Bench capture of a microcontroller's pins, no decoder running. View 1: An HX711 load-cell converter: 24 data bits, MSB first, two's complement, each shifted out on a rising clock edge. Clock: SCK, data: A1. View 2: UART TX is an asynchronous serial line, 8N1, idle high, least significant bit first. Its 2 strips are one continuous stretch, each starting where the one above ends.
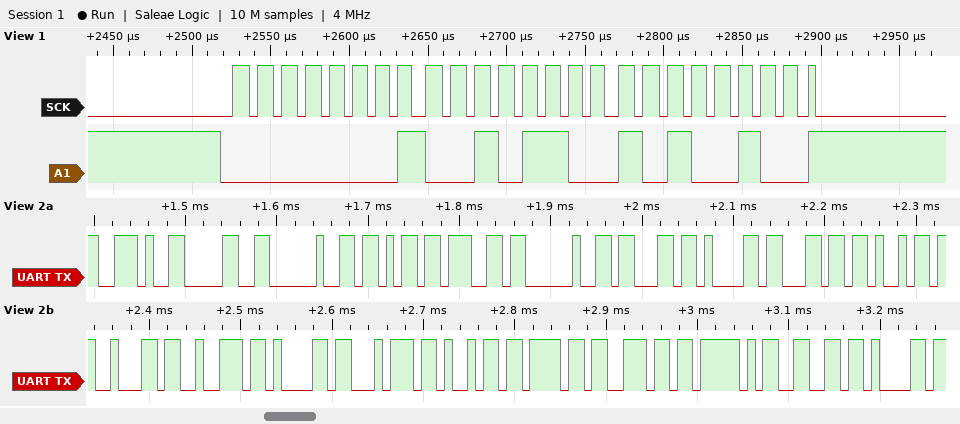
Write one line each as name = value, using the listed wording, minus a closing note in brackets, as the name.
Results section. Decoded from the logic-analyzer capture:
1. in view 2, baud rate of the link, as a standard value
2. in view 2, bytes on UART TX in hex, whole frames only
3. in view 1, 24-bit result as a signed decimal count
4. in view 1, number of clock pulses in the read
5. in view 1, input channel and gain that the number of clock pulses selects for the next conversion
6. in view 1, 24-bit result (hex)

in view 2, baud rate of the link, as a standard value = 115200 baud
in view 2, bytes on UART TX in hex, whole frames only = 0x2E 0x30 0x20 0x6B 0x67 0x20 0x63 0x61 0x6C 0x69 0x62 0x72 0x61 0x74 0x69 0x6F 0x6E 0x5F 0x66 0x61
in view 1, 24-bit result as a signed decimal count = 76964
in view 1, number of clock pulses in the read = 25
in view 1, input channel and gain that the number of clock pulses selects for the next conversion = channel A, gain 128
in view 1, 24-bit result = 0x012CA4
